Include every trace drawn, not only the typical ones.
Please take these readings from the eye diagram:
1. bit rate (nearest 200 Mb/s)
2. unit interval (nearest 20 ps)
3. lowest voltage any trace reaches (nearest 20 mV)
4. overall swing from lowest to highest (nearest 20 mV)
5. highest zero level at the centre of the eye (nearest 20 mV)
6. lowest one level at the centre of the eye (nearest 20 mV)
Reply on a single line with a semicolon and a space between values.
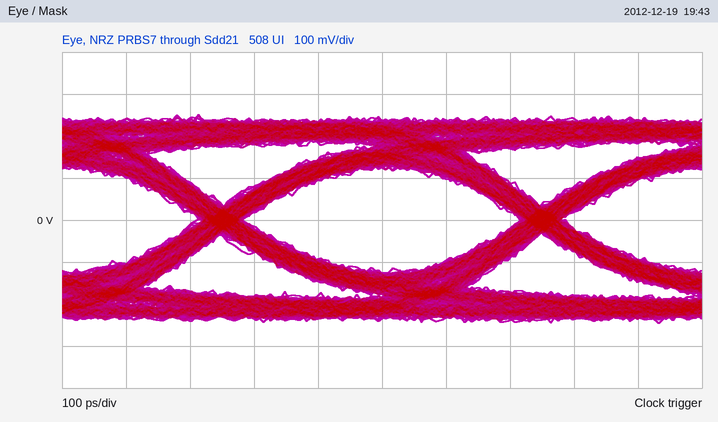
2.0 Gb/s; 500 ps; -240 mV; 500 mV; -120 mV; 120 mV
